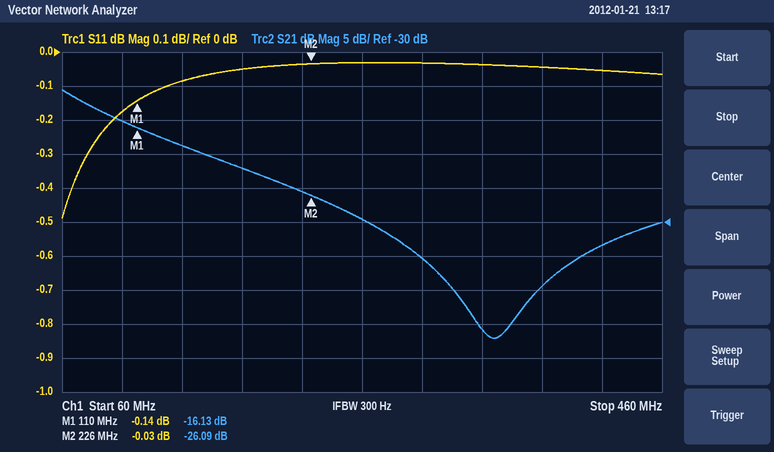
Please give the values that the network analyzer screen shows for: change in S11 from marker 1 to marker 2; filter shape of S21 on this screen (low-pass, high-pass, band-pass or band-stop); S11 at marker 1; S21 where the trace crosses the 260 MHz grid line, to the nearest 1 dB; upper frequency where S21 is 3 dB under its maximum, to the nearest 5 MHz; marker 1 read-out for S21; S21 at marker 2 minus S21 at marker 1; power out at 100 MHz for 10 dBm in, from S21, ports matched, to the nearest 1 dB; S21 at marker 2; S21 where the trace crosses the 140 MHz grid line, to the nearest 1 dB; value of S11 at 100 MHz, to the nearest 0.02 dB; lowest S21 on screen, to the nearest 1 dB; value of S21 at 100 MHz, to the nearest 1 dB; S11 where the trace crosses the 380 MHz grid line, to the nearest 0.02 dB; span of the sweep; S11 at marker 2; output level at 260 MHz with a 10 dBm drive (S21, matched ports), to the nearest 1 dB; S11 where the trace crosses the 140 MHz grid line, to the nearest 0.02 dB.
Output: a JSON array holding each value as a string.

["0.11 dB", "low-pass", "-0.14 dB", "-30 dB", "85 MHz", "-16.13 dB", "-9.96 dB", "-5 dBm", "-26.09 dB", "-19 dB", "-0.18 dB", "-47 dB", "-15 dB", "-0.04 dB", "400 MHz", "-0.03 dB", "-20 dBm", "-0.08 dB"]
